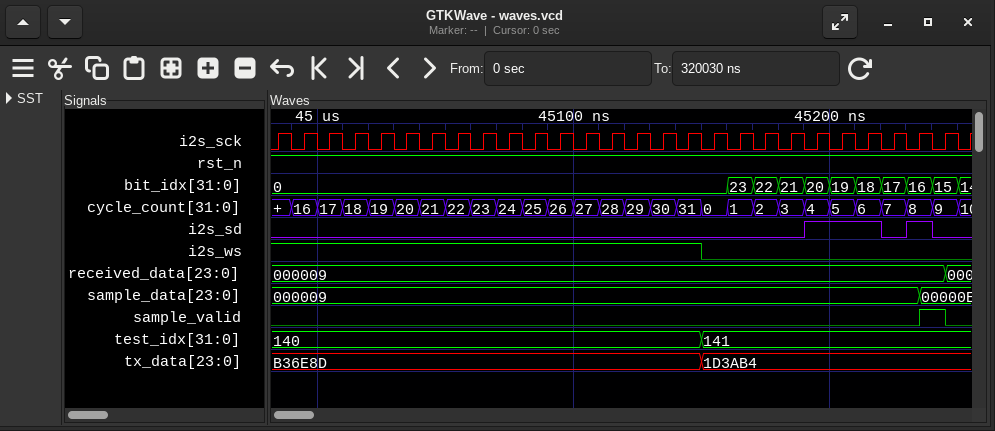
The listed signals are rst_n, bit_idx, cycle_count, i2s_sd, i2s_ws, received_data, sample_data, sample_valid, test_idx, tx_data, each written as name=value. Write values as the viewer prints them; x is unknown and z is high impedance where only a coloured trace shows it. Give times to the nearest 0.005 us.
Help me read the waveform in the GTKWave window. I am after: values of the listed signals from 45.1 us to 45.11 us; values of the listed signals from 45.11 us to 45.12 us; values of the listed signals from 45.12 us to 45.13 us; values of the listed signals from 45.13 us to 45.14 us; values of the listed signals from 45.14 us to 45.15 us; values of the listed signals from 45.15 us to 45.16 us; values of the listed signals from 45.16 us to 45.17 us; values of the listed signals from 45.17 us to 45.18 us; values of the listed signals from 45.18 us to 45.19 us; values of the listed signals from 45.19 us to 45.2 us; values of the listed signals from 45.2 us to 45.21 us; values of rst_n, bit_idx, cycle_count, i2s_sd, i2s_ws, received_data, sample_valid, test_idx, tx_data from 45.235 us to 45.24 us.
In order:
rst_n=1, bit_idx=0, cycle_count=27, i2s_sd=0, i2s_ws=1, received_data=000009, sample_data=000009, sample_valid=0, test_idx=140, tx_data=B36E8D
rst_n=1, bit_idx=0, cycle_count=28, i2s_sd=0, i2s_ws=1, received_data=000009, sample_data=000009, sample_valid=0, test_idx=140, tx_data=B36E8D
rst_n=1, bit_idx=0, cycle_count=29, i2s_sd=0, i2s_ws=1, received_data=000009, sample_data=000009, sample_valid=0, test_idx=140, tx_data=B36E8D
rst_n=1, bit_idx=0, cycle_count=30, i2s_sd=0, i2s_ws=1, received_data=000009, sample_data=000009, sample_valid=0, test_idx=140, tx_data=B36E8D
rst_n=1, bit_idx=0, cycle_count=31, i2s_sd=0, i2s_ws=1, received_data=000009, sample_data=000009, sample_valid=0, test_idx=140, tx_data=B36E8D
rst_n=1, bit_idx=0, cycle_count=0, i2s_sd=0, i2s_ws=0, received_data=000009, sample_data=000009, sample_valid=0, test_idx=141, tx_data=1D3AB4
rst_n=1, bit_idx=23, cycle_count=1, i2s_sd=0, i2s_ws=0, received_data=000009, sample_data=000009, sample_valid=0, test_idx=141, tx_data=1D3AB4
rst_n=1, bit_idx=22, cycle_count=2, i2s_sd=0, i2s_ws=0, received_data=000009, sample_data=000009, sample_valid=0, test_idx=141, tx_data=1D3AB4
rst_n=1, bit_idx=21, cycle_count=3, i2s_sd=0, i2s_ws=0, received_data=000009, sample_data=000009, sample_valid=0, test_idx=141, tx_data=1D3AB4
rst_n=1, bit_idx=20, cycle_count=4, i2s_sd=1, i2s_ws=0, received_data=000009, sample_data=000009, sample_valid=0, test_idx=141, tx_data=1D3AB4
rst_n=1, bit_idx=19, cycle_count=5, i2s_sd=1, i2s_ws=0, received_data=000009, sample_data=000009, sample_valid=0, test_idx=141, tx_data=1D3AB4
rst_n=1, bit_idx=16, cycle_count=8, i2s_sd=1, i2s_ws=0, received_data=000009, sample_valid=1, test_idx=141, tx_data=1D3AB4
